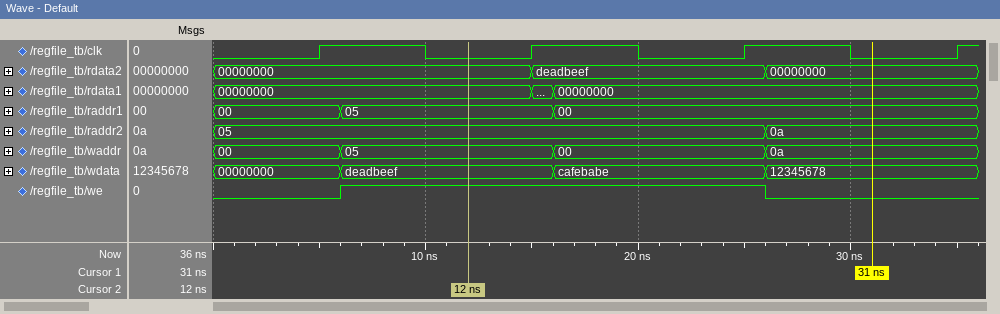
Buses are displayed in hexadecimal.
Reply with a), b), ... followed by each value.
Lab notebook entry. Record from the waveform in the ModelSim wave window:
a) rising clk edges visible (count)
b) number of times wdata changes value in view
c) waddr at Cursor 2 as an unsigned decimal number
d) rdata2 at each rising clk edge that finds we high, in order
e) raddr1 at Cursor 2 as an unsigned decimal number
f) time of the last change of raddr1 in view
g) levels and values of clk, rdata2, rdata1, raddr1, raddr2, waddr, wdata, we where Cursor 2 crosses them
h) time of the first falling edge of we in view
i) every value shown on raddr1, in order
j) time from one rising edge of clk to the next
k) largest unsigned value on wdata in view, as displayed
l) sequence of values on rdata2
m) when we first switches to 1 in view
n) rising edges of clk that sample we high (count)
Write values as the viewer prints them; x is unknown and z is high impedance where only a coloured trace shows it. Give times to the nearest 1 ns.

a) 4
b) 3
c) 5
d) 00000000, deadbeef
e) 5
f) 16 ns
g) clk=0, rdata2=00000000, rdata1=00000000, raddr1=05, raddr2=05, waddr=05, wdata=deadbeef, we=1
h) 26 ns
i) 00, 05, 00
j) 10 ns
k) deadbeef
l) 00000000, deadbeef, 00000000
m) 6 ns
n) 2
